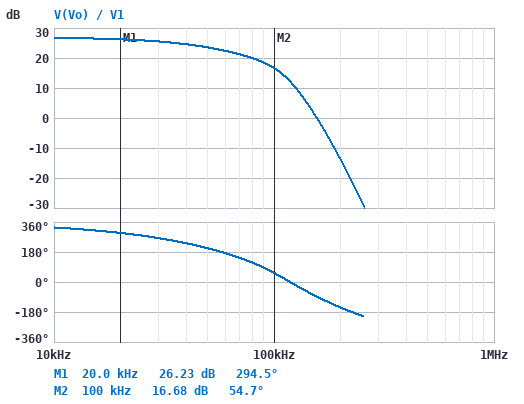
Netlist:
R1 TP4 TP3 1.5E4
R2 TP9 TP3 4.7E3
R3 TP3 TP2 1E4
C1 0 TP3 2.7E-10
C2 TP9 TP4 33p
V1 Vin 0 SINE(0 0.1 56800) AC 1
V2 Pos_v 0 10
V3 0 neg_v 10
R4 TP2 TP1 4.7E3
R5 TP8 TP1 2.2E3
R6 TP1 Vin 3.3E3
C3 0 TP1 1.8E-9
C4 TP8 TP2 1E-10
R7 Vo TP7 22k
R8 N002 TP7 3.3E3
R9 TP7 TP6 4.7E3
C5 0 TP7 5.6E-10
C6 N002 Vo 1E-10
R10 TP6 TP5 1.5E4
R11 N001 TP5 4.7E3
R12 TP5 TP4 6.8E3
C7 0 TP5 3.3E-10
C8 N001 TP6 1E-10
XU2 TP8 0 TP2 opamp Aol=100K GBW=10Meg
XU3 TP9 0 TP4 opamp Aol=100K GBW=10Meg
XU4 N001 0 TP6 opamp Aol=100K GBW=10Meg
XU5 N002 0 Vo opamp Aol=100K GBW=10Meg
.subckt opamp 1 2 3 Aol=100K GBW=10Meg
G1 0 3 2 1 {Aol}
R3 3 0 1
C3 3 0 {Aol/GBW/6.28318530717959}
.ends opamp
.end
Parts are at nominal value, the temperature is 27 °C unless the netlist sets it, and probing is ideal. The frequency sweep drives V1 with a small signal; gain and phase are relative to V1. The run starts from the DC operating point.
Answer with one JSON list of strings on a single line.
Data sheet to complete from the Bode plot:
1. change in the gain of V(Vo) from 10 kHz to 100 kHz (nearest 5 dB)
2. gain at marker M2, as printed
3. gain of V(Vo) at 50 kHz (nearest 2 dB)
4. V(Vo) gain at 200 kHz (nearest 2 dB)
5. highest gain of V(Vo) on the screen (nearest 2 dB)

["-10 dB", "16.68 dB", "24 dB", "-14 dB", "26 dB"]
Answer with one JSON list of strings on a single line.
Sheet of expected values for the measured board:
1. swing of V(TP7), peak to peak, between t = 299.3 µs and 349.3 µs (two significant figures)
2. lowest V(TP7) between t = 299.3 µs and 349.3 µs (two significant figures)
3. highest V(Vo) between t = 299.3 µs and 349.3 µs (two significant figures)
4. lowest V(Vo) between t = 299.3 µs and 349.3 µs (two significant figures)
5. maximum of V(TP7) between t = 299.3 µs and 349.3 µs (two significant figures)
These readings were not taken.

["340 mV", "-170 mV", "1.4 V", "-1.4 V", "170 mV"]
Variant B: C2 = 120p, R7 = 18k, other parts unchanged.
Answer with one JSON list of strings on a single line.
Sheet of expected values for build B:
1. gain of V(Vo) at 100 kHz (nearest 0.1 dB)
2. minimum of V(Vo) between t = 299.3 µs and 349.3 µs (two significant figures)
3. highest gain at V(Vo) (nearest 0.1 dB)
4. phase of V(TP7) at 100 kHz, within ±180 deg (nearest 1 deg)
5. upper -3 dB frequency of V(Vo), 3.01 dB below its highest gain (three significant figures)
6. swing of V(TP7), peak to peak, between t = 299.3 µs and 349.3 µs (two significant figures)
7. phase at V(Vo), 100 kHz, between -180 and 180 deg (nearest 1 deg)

["9.8 dB", "-920 mV", "25.1 dB", "-80 deg", "39.3 kHz", "230 mV", "10 deg"]
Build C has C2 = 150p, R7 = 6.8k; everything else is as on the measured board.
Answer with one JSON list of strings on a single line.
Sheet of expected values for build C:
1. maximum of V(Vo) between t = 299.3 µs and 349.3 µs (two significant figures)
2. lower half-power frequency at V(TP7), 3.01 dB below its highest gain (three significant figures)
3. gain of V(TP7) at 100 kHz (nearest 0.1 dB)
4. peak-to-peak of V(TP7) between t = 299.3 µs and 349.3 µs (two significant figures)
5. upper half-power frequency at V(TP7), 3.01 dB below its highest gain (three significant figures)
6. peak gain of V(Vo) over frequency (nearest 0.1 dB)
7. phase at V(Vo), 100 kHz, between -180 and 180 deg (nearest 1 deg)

["410 mV", "29.4 kHz", "-7.5 dB", "100 mV", "108 kHz", "16.7 dB", "41 deg"]
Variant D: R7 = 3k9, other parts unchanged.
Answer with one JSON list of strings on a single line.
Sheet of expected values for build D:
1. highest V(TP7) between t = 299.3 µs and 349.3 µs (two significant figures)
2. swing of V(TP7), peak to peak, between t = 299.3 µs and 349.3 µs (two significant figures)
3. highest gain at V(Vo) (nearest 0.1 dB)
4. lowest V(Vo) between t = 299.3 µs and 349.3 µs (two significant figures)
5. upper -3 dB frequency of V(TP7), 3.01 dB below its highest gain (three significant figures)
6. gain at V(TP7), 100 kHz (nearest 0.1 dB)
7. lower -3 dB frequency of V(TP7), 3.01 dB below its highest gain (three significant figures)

["48 mV", "96 mV", "11.8 dB", "-390 mV", "131 kHz", "-2.5 dB", "62.8 kHz"]
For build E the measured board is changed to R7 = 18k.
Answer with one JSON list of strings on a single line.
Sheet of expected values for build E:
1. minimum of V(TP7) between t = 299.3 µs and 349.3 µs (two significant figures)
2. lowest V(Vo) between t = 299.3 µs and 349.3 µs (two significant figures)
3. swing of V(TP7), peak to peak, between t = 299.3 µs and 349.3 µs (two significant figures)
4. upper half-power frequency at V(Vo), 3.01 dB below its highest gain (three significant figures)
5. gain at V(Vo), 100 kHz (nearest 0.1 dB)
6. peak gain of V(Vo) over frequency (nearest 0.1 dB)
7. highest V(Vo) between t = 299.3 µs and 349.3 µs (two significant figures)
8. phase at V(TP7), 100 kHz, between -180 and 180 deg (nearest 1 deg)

["-160 mV", "-1.3 V", "320 mV", "57.7 kHz", "16.7 dB", "25.1 dB", "1.3 V", "-30 deg"]
